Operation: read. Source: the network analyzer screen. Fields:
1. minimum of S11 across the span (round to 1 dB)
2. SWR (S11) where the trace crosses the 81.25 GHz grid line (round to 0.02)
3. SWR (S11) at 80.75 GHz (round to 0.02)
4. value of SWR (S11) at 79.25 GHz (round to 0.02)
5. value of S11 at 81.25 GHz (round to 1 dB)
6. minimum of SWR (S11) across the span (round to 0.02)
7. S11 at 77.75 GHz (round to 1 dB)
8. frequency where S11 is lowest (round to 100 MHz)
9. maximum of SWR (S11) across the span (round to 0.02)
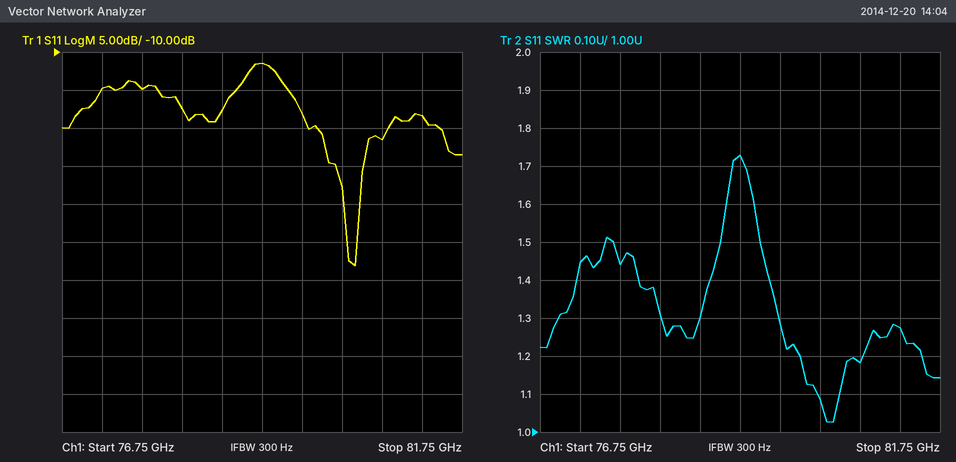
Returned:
-38 dB
1.28
1.18
1.72
-18 dB
1.02
-15 dB
80.4 GHz
1.72
